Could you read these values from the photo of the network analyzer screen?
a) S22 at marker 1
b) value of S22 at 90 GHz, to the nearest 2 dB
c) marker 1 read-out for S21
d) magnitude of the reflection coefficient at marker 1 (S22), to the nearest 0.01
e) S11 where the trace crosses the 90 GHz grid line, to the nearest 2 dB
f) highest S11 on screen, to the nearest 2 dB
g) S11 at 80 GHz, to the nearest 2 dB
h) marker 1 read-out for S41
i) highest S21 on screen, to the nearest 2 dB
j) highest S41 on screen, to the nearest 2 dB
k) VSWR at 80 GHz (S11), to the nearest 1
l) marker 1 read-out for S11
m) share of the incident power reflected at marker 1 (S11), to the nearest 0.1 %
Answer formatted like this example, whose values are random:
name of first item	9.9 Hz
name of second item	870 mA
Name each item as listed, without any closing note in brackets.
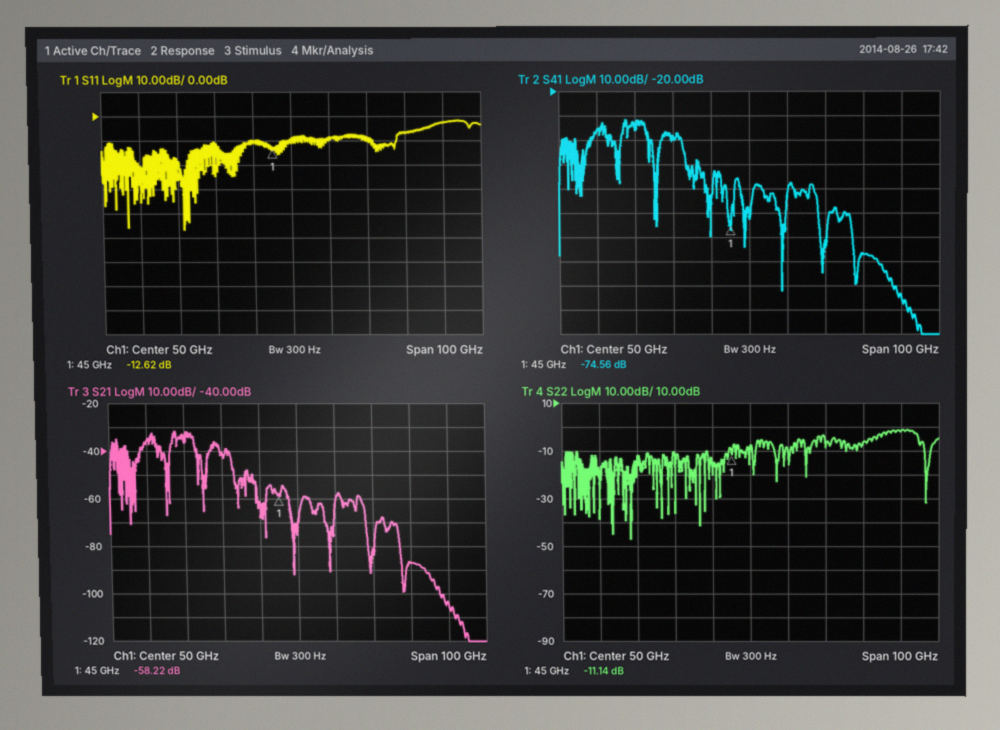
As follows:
S22 at marker 1	-11.14 dB
value of S22 at 90 GHz, to the nearest 2 dB	-2 dB
marker 1 read-out for S21	-58.22 dB
magnitude of the reflection coefficient at marker 1 (S22), to the nearest 0.01	0.28
S11 where the trace crosses the 90 GHz grid line, to the nearest 2 dB	-2 dB
highest S11 on screen, to the nearest 2 dB	-2 dB
S11 at 80 GHz, to the nearest 2 dB	-6 dB
marker 1 read-out for S41	-74.56 dB
highest S21 on screen, to the nearest 2 dB	-32 dB
highest S41 on screen, to the nearest 2 dB	-32 dB
VSWR at 80 GHz (S11), to the nearest 1	3
marker 1 read-out for S11	-12.62 dB
share of the incident power reflected at marker 1 (S11), to the nearest 0.1 %	5.5 %
